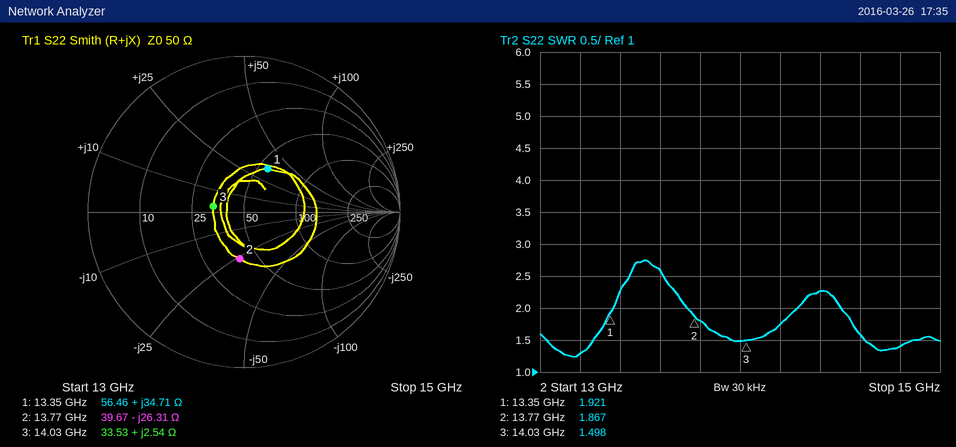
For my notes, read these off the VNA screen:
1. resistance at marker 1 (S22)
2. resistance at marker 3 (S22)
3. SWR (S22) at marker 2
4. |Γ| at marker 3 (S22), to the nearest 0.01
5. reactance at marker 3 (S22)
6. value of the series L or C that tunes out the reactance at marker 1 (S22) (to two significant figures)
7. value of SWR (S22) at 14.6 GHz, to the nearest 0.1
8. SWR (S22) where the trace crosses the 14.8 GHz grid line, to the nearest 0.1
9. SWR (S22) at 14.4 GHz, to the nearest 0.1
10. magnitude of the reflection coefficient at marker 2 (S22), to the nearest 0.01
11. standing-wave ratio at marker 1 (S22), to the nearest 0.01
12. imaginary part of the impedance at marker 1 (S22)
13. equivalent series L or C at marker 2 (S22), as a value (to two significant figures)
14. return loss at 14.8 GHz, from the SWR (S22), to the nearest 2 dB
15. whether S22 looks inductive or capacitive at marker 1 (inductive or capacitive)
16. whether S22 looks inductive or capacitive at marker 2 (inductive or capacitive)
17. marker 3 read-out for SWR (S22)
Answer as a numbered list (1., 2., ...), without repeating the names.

1. 56.46 Ω
2. 33.53 Ω
3. 1.867
4. 0.20
5. +2.54 Ω
6. 340 fF
7. 1.6
8. 1.4
9. 2.3
10. 0.30
11. 1.92
12. +34.71 Ω
13. 440 fF
14. 16 dB
15. inductive
16. capacitive
17. 1.498
